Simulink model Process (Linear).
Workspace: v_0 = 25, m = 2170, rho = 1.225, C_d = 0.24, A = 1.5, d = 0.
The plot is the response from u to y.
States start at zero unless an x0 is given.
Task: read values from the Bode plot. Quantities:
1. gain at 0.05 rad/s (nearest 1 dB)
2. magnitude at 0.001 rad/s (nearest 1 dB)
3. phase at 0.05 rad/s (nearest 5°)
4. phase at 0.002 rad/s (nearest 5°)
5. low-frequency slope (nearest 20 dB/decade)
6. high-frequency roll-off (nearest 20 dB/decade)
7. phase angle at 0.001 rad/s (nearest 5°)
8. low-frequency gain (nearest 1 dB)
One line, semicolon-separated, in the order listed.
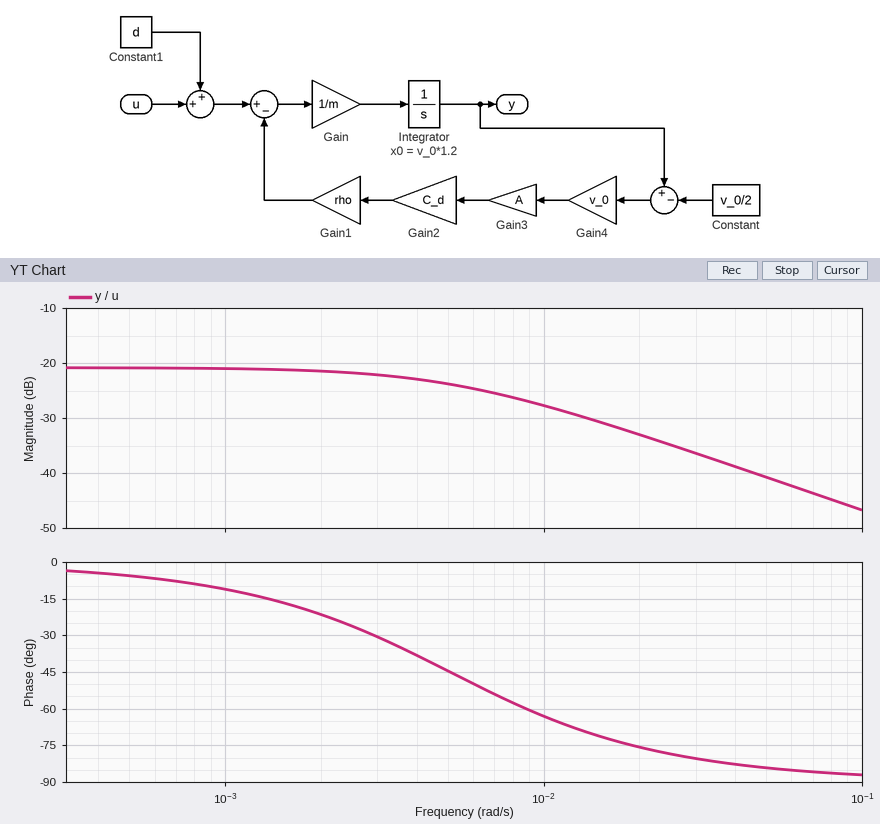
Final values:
-41 dB; -21 dB; -85°; -20°; 0 dB/decade; -20 dB/decade; -10°; -21 dB
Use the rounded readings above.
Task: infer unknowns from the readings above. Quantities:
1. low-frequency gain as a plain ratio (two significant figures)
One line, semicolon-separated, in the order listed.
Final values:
0.089
